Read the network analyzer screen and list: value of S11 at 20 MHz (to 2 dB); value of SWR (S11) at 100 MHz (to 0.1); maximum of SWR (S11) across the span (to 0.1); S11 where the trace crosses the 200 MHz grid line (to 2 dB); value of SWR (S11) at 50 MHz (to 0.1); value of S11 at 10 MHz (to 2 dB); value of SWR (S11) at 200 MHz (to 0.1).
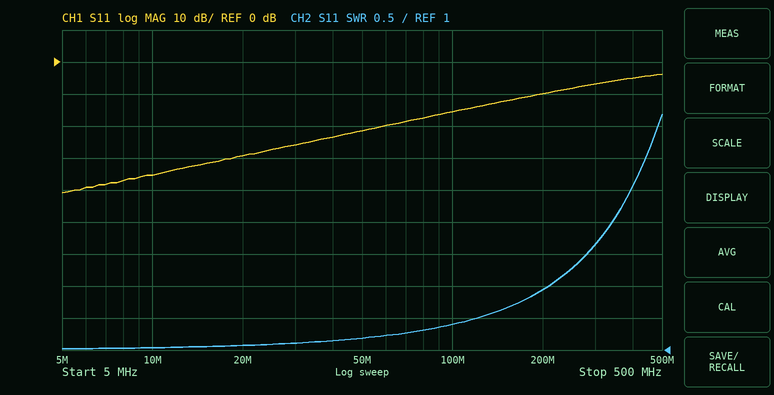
-30 dB
1.4
4.7
-10 dB
1.2
-36 dB
1.9
